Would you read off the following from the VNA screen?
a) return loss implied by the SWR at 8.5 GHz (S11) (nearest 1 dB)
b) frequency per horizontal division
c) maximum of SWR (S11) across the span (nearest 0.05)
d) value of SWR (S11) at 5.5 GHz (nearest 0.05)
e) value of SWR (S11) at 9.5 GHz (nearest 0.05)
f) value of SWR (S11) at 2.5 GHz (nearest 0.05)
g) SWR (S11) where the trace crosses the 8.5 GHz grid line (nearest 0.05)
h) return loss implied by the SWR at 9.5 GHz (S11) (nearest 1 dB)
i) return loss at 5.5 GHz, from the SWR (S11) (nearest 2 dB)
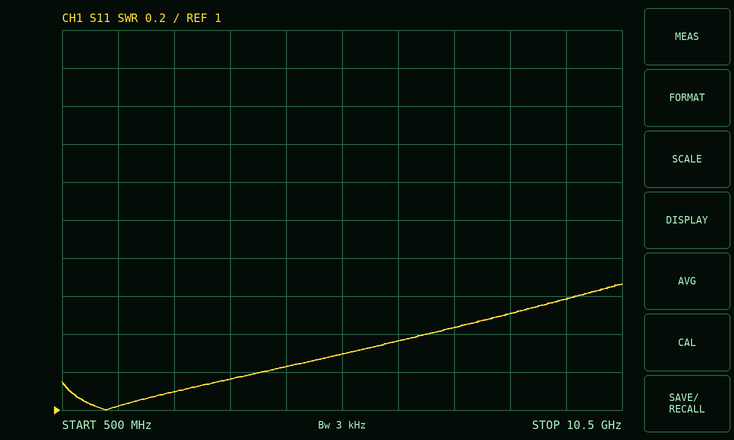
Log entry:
14 dB
1 GHz
1.65
1.30
1.60
1.10
1.50
13 dB
18 dB
